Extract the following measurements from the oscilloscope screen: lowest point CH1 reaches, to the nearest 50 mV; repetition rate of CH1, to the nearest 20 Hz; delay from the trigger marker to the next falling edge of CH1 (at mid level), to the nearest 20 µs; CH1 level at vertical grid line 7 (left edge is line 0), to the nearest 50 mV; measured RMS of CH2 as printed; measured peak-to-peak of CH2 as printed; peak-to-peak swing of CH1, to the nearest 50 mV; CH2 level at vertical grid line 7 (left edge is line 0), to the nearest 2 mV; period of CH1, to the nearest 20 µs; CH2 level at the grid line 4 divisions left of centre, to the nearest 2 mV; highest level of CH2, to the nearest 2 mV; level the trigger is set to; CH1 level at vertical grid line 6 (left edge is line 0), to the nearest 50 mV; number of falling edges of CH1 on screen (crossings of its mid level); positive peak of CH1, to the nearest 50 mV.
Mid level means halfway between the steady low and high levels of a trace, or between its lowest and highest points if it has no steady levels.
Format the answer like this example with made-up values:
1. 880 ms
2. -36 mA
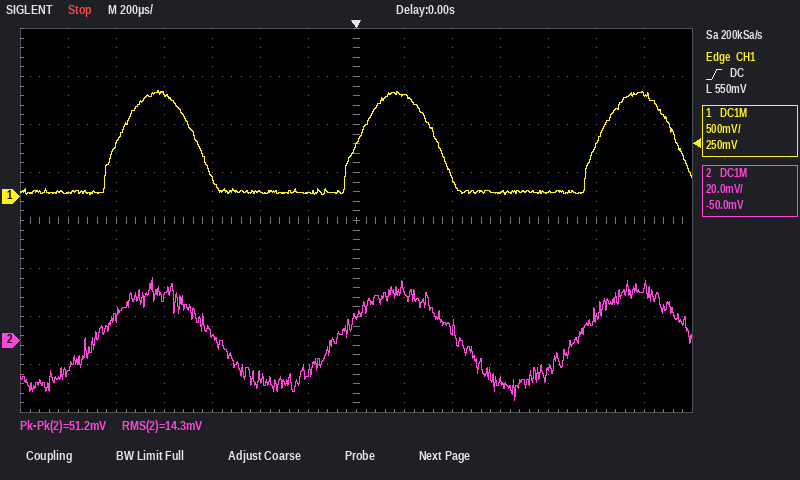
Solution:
1. 0 mV
2. 1.00 kHz
3. 340 µs
4. 550 mV
5. 14.3 mV
6. 51.2 mV
7. 1.10 V
8. 10 mV
9. 1.00 ms
10. 18 mV
11. 26 mV
12. 550 mV
13. 50 mV
14. 3
15. 1.10 V
